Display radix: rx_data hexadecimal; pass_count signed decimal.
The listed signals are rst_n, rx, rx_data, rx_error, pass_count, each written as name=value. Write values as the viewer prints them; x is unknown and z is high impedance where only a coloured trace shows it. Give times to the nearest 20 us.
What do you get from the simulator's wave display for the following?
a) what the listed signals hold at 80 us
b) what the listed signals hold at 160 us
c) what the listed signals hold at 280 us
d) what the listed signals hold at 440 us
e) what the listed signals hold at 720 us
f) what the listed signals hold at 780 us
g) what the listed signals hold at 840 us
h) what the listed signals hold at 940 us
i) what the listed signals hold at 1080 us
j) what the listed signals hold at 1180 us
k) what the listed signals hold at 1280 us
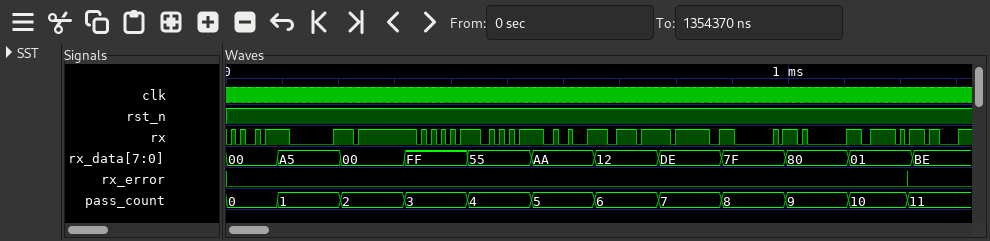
rst_n=1, rx=1, rx_data=00, rx_error=0, pass_count=0
rst_n=1, rx=0, rx_data=A5, rx_error=0, pass_count=1
rst_n=1, rx=1, rx_data=00, rx_error=0, pass_count=2
rst_n=1, rx=1, rx_data=55, rx_error=0, pass_count=4
rst_n=1, rx=1, rx_data=12, rx_error=0, pass_count=6
rst_n=1, rx=1, rx_data=DE, rx_error=0, pass_count=7
rst_n=1, rx=1, rx_data=DE, rx_error=0, pass_count=7
rst_n=1, rx=0, rx_data=7F, rx_error=0, pass_count=8
rst_n=1, rx=0, rx_data=80, rx_error=0, pass_count=9
rst_n=1, rx=1, rx_data=01, rx_error=0, pass_count=10
rst_n=1, rx=0, rx_data=BE, rx_error=0, pass_count=11
